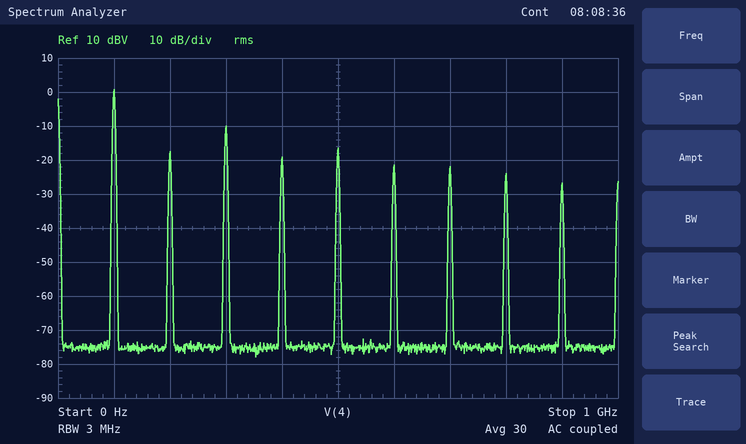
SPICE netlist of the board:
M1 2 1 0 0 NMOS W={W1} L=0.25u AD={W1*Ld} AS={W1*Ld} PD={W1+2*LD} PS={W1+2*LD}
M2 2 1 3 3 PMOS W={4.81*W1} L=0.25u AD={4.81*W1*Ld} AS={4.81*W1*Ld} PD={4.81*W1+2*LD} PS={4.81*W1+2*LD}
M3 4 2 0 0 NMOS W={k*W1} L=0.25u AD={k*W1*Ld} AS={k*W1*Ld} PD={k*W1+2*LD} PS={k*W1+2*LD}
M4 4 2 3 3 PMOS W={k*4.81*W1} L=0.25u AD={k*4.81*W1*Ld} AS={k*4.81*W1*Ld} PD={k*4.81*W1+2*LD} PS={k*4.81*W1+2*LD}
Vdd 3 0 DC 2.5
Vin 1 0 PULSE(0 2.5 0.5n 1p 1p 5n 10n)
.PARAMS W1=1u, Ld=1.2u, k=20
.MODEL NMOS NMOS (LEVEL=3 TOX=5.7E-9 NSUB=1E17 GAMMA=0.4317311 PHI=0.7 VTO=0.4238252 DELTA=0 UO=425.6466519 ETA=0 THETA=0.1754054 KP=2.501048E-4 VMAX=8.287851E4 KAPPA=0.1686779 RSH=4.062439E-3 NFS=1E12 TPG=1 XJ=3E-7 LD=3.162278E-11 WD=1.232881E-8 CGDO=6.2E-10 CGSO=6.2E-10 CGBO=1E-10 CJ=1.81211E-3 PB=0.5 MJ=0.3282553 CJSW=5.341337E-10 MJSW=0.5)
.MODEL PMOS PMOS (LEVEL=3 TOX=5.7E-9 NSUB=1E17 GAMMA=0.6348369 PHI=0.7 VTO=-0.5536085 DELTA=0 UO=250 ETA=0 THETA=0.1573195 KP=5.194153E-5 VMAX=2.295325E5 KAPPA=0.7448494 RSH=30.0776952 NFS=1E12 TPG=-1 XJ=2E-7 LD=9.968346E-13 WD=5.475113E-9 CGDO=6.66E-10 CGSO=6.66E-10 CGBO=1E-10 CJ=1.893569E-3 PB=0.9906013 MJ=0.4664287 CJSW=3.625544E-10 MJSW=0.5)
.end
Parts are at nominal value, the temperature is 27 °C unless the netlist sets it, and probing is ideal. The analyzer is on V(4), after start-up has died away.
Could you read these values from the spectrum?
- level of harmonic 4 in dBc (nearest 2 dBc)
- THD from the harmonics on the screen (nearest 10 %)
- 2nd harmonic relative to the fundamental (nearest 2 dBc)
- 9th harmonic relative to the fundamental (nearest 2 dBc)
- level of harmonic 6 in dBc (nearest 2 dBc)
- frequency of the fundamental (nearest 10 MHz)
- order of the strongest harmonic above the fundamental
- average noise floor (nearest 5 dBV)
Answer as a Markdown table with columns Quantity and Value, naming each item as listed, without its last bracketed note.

| Quantity | Value |
|---|---|
| level of harmonic 4 in dBc | -20 dBc |
| THD from the harmonics on the screen | 40 % |
| 2nd harmonic relative to the fundamental | -18 dBc |
| 9th harmonic relative to the fundamental | -28 dBc |
| level of harmonic 6 in dBc | -22 dBc |
| frequency of the fundamental | 100 MHz |
| order of the strongest harmonic above the fundamental | 3 |
| average noise floor | -75 dBV |
